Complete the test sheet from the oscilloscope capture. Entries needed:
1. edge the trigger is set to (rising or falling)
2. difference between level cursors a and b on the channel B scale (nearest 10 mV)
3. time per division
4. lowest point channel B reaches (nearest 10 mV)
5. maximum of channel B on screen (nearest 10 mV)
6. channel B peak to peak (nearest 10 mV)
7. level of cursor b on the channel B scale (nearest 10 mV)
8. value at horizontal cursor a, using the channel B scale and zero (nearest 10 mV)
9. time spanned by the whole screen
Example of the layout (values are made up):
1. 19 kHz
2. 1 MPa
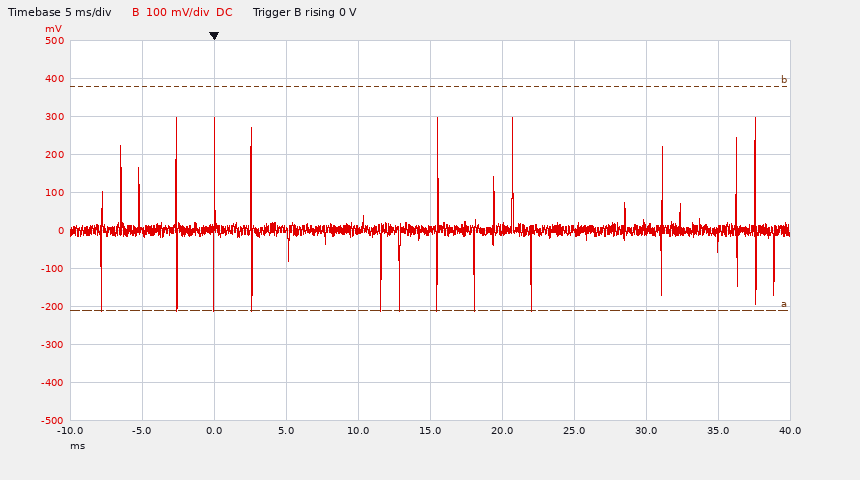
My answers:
1. rising
2. 590 mV
3. 5 ms
4. -210 mV
5. 300 mV
6. 510 mV
7. 380 mV
8. -210 mV
9. 50 ms
